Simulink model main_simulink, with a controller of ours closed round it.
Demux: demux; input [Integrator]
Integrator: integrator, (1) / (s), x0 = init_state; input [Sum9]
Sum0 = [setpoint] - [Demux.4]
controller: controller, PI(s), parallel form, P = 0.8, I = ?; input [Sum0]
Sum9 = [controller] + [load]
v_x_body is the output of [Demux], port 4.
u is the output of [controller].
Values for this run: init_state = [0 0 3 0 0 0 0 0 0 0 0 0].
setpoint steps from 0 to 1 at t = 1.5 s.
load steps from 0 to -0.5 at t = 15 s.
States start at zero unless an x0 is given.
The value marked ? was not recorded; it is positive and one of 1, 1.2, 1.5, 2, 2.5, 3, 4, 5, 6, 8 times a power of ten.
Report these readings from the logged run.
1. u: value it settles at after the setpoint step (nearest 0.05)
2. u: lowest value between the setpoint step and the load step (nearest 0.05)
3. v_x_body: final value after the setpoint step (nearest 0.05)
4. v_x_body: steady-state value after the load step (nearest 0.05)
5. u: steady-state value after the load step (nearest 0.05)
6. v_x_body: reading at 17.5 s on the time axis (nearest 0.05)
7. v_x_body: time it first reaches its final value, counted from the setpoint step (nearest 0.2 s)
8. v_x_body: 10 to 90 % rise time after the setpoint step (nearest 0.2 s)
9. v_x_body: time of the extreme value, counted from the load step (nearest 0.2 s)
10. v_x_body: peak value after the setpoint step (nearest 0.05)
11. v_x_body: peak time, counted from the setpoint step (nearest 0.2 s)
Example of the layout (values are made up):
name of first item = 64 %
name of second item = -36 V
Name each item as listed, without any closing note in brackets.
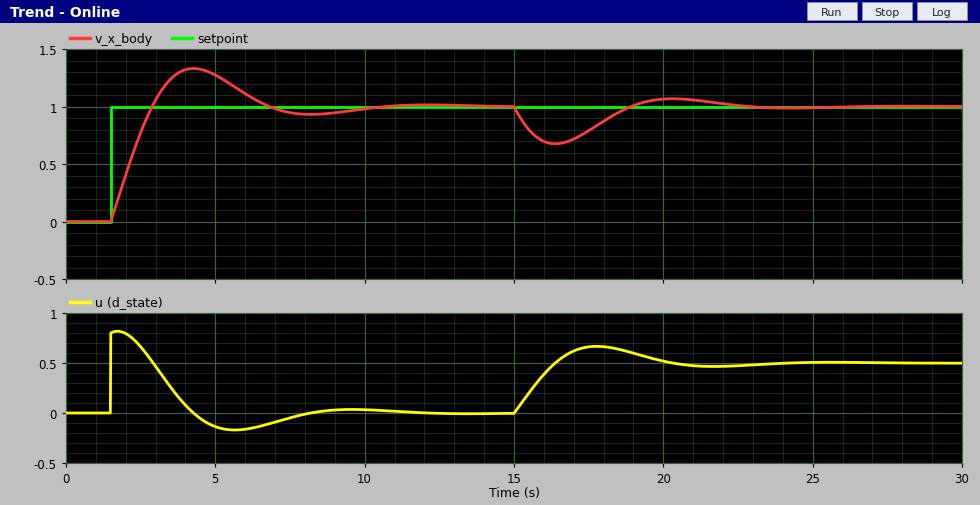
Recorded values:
u: value it settles at after the setpoint step = 0.00
u: lowest value between the setpoint step and the load step = -0.15
v_x_body: final value after the setpoint step = 1.00
v_x_body: steady-state value after the load step = 1.00
u: steady-state value after the load step = 0.50
v_x_body: reading at 17.5 s on the time axis = 0.80
v_x_body: time it first reaches its final value, counted from the setpoint step = 1.4 s
v_x_body: 10 to 90 % rise time after the setpoint step = 1.0 s
v_x_body: time of the extreme value, counted from the load step = 1.4 s
v_x_body: peak value after the setpoint step = 1.35
v_x_body: peak time, counted from the setpoint step = 2.8 s
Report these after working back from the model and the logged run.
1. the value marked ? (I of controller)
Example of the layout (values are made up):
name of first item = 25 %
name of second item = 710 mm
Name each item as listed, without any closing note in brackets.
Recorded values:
the value marked ? = 0.8
